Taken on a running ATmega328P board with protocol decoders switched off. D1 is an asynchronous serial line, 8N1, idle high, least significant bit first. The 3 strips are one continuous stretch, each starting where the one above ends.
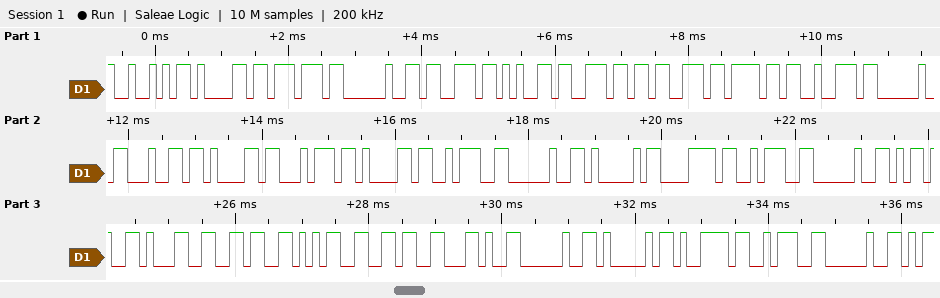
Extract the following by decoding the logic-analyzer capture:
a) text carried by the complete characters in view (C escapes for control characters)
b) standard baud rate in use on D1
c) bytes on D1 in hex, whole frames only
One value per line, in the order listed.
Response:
"Raw sensor data: Ax: -1656, Ay: "
9600 baud
52 61 77 20 73 65 6E 73 6F 72 20 64 61 74 61 3A 20 41 78 3A 20 2D 31 36 35 36 2C 20 41 79 3A 20
